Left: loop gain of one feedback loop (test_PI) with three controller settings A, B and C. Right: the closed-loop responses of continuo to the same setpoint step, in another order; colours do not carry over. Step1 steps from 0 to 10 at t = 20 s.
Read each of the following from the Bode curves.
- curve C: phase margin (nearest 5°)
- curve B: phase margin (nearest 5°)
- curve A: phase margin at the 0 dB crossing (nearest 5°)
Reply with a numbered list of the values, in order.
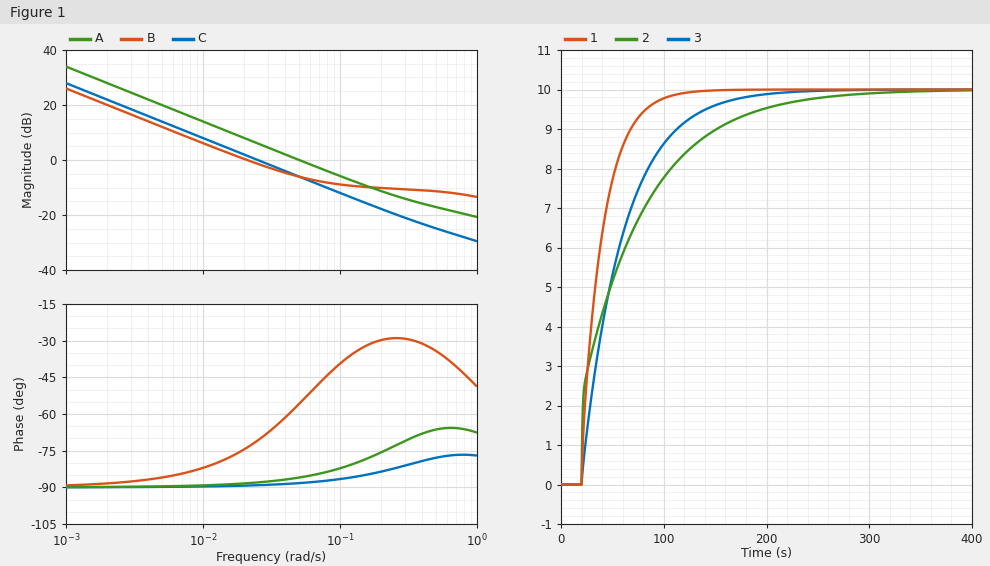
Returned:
1. 90°
2. 105°
3. 95°
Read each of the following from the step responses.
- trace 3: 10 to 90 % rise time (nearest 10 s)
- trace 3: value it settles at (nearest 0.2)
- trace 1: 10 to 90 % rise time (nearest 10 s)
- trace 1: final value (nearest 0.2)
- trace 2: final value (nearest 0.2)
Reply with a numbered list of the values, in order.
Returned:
1. 90 s
2. 10.0
3. 50 s
4. 10.0
5. 10.0
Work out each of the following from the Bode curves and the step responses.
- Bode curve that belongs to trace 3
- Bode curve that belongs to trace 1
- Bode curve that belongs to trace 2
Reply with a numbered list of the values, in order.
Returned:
1. C
2. A
3. B
